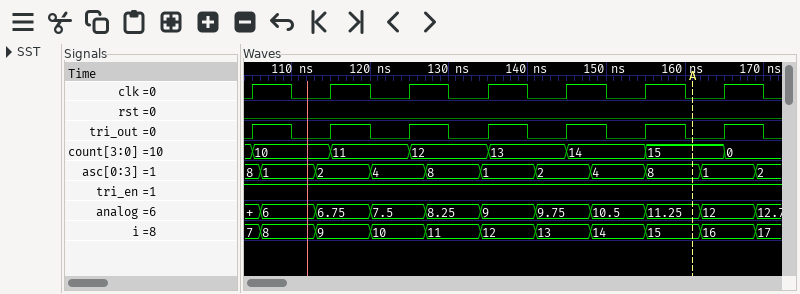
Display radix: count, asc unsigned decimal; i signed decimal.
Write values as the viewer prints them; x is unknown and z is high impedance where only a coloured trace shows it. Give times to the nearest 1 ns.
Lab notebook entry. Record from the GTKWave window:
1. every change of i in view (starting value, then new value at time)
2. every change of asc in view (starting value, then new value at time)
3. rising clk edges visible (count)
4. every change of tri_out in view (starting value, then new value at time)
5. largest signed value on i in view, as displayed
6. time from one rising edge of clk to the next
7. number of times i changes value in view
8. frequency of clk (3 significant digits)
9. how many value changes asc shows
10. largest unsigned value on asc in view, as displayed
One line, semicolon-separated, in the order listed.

7, 8 at 106 ns, 9 at 113 ns, 10 at 120 ns, 11 at 127 ns, 12 at 134 ns, 13 at 141 ns, 14 at 148 ns, 15 at 155 ns, 16 at 162 ns, 17 at 169 ns; 8, 1 at 106 ns, 2 at 113 ns, 4 at 120 ns, 8 at 127 ns, 1 at 134 ns, 2 at 141 ns, 4 at 148 ns, 8 at 155 ns, 1 at 162 ns, 2 at 169 ns; 7; 0, 1 at 105 ns, 0 at 110 ns, 1 at 115 ns, 0 at 120 ns, 1 at 125 ns, 0 at 130 ns, 1 at 135 ns, 0 at 140 ns, 1 at 145 ns, 0 at 150 ns, 1 at 155 ns, 0 at 160 ns, 1 at 165 ns, 0 at 170 ns; 17; 10 ns; 10; 100 MHz; 10; 8
